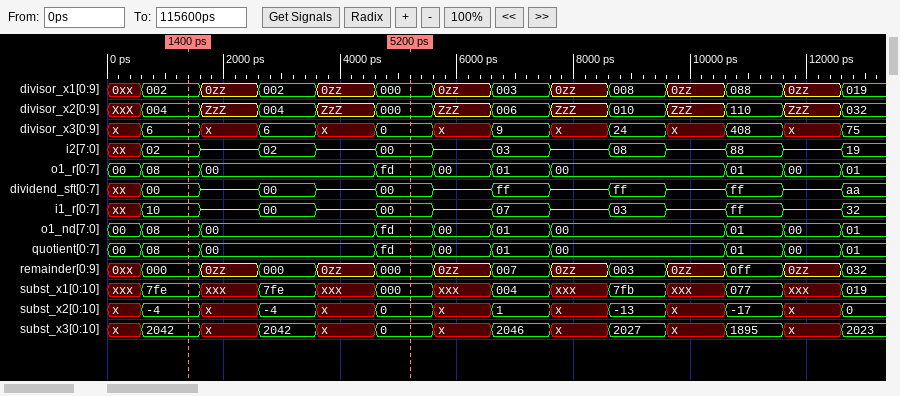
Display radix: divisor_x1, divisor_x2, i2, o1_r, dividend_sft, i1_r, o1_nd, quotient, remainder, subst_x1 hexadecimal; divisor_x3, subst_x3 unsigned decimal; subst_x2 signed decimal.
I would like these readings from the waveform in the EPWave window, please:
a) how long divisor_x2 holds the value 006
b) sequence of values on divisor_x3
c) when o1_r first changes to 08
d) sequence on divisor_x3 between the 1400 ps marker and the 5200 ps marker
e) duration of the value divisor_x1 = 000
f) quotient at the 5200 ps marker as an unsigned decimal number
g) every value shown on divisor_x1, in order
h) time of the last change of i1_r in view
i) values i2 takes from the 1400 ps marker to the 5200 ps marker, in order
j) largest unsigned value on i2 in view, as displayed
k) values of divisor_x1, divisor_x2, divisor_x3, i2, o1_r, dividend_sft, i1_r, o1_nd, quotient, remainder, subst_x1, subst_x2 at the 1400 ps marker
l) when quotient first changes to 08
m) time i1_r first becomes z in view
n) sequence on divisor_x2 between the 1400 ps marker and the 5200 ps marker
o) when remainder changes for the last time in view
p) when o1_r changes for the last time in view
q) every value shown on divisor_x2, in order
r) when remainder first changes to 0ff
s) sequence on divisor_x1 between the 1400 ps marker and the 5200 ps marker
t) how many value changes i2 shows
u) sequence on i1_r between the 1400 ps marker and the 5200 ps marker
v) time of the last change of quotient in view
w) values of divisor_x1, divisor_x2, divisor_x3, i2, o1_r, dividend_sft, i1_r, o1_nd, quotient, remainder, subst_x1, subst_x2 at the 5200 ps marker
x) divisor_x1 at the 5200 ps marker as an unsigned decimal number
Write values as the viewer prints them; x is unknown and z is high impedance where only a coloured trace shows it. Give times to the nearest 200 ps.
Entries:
1000 ps
x, 6, x, 6, x, 0, x, 9, x, 24, x, 408, x, 75
600 ps
6, x, 6, x, 0
1000 ps
253
0xx, 002, 0zz, 002, 0zz, 000, 0zz, 003, 0zz, 008, 0zz, 088, 0zz, 019
12600 ps
02, z, 02, z, 00
88
divisor_x1=002, divisor_x2=004, divisor_x3=6, i2=02, o1_r=08, dividend_sft=00, i1_r=10, o1_nd=08, quotient=08, remainder=000, subst_x1=7fe, subst_x2=-4
600 ps
1600 ps
004, ZzZ, 004, ZzZ, 000
12600 ps
12600 ps
XxX, 004, ZzZ, 004, ZzZ, 000, ZzZ, 006, ZzZ, 010, ZzZ, 110, ZzZ, 032
10600 ps
002, 0zz, 002, 0zz, 000
13
10, z, 00, z, 00
12600 ps
divisor_x1=000, divisor_x2=000, divisor_x3=0, i2=00, o1_r=fd, dividend_sft=00, i1_r=00, o1_nd=fd, quotient=fd, remainder=000, subst_x1=000, subst_x2=0
0
